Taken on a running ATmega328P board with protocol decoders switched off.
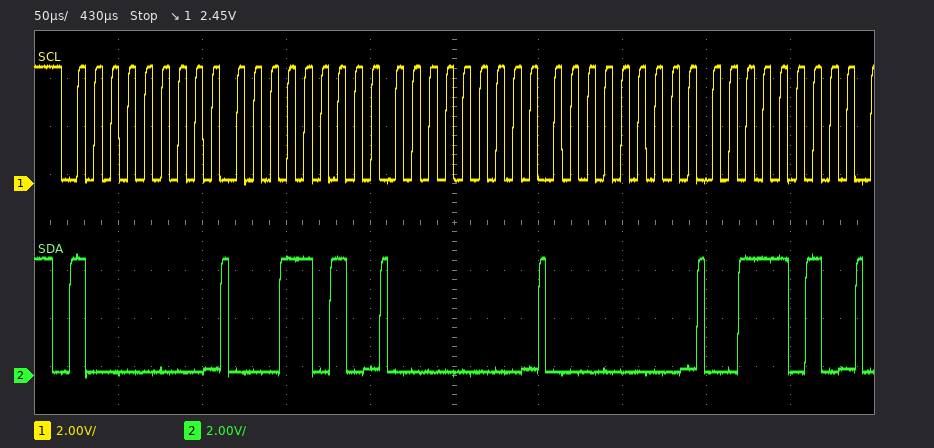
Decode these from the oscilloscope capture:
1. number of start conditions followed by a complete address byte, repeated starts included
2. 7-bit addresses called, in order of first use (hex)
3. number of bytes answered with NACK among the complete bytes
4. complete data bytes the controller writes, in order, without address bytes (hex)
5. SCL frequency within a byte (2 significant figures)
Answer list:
1
0x40
0
1A 00 00 3A
100 kHz
